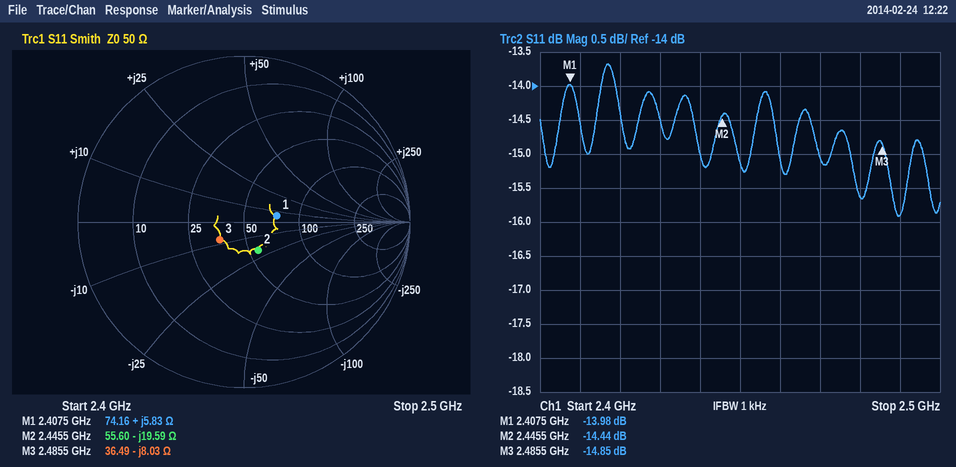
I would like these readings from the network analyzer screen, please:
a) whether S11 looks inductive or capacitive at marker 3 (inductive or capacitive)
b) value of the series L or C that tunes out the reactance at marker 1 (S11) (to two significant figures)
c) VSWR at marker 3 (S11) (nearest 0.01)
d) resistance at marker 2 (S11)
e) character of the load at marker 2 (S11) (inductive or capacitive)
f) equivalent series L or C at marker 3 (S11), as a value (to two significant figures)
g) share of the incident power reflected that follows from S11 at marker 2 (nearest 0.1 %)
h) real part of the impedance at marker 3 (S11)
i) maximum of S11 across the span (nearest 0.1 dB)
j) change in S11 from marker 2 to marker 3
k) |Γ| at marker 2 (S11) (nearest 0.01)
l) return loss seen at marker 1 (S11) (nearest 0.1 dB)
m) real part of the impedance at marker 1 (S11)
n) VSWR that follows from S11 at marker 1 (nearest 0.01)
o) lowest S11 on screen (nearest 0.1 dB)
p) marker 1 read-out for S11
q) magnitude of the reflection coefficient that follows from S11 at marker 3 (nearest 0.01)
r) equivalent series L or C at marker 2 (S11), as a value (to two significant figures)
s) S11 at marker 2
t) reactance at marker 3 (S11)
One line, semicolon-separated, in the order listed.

capacitive; 11 pF; 1.44; 55.60 Ω; capacitive; 8.0 pF; 3.6 %; 36.49 Ω; -13.7 dB; -0.41 dB; 0.19; 14.0 dB; 74.16 Ω; 1.50; -15.9 dB; -13.98 dB; 0.18; 3.3 pF; -14.44 dB; -8.03 Ω
